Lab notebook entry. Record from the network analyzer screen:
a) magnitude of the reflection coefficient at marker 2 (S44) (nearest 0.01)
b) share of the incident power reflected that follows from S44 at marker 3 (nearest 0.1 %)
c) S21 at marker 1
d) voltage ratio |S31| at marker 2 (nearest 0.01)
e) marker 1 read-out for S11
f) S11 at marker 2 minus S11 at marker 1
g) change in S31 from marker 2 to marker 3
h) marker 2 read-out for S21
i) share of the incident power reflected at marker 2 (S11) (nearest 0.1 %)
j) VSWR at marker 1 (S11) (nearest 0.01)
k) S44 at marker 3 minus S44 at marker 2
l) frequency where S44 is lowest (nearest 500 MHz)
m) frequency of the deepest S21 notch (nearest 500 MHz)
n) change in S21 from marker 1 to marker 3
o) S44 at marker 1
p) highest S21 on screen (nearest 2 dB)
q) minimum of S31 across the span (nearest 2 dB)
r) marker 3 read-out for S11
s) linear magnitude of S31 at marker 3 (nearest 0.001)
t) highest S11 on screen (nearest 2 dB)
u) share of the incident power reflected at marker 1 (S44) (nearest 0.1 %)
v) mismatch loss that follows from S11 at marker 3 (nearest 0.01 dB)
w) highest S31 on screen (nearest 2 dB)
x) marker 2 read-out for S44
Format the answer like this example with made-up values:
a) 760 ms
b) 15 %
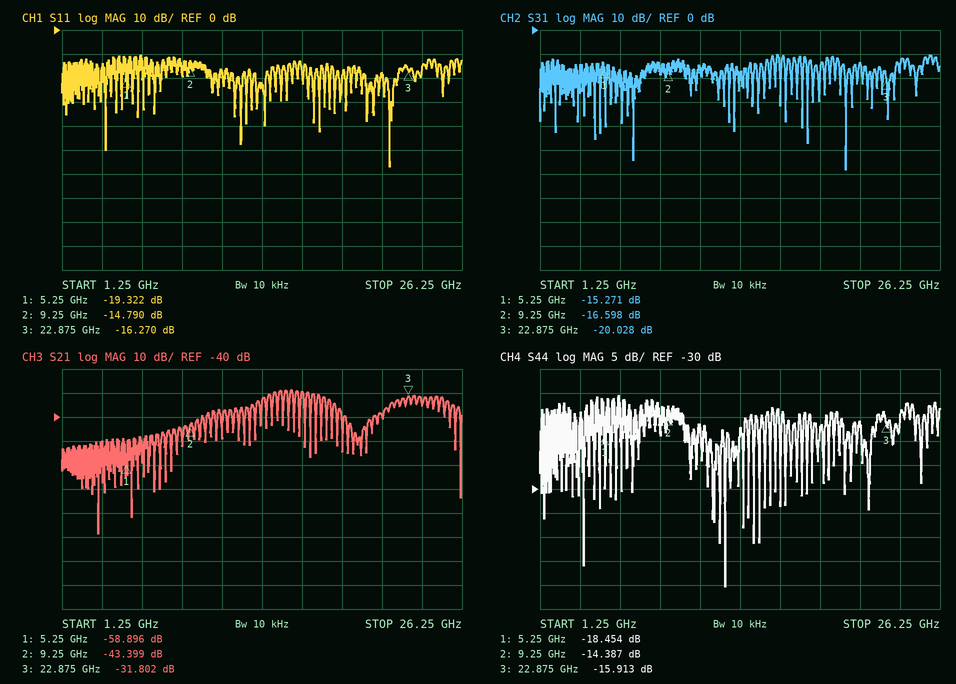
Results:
a) 0.19
b) 2.6 %
c) -58.896 dB
d) 0.15
e) -19.322 dB
f) 4.532 dB
g) -3.430 dB
h) -43.399 dB
i) 3.3 %
j) 1.24
k) -1.526 dB
l) 13.0 GHz
m) 3.5 GHz
n) 27.094 dB
o) -18.454 dB
p) -28 dB
q) -58 dB
r) -16.270 dB
s) 0.100
t) -10 dB
u) 1.4 %
v) 0.10 dB
w) -10 dB
x) -14.387 dB
